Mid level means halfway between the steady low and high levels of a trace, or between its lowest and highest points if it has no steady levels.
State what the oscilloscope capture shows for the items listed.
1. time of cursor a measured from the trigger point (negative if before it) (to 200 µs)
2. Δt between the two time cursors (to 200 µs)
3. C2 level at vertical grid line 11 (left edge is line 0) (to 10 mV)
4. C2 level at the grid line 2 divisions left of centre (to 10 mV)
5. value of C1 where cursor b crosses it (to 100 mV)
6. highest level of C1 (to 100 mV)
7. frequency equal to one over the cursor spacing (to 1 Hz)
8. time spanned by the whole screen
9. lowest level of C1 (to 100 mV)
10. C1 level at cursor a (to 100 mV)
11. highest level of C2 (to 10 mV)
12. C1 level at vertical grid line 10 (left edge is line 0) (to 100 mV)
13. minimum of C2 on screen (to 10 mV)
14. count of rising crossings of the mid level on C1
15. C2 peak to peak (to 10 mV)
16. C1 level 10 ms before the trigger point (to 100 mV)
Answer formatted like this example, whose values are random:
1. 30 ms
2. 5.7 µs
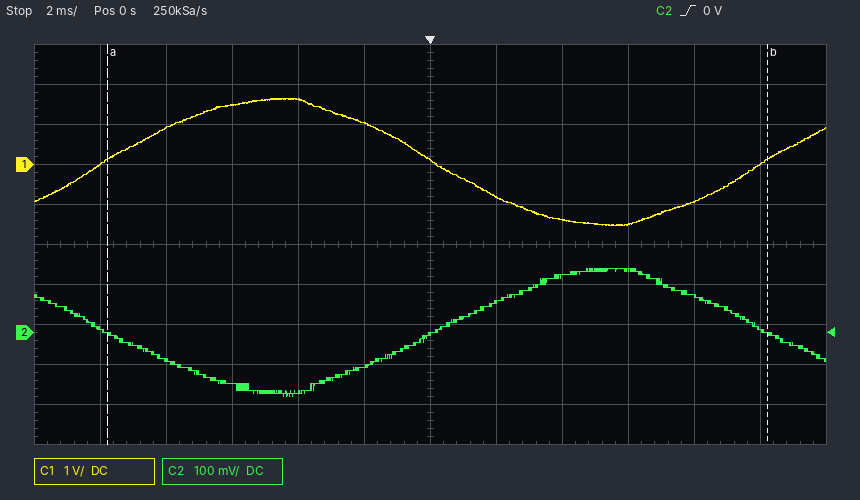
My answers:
1. -9.8 ms
2. 20.0 ms
3. 10 mV
4. -150 mV
5. 100 mV
6. 1.6 V
7. 50 Hz
8. 24 ms
9. -1.5 V
10. 100 mV
11. 160 mV
12. -900 mV
13. -160 mV
14. 2
15. 320 mV
16. 0.0 V
